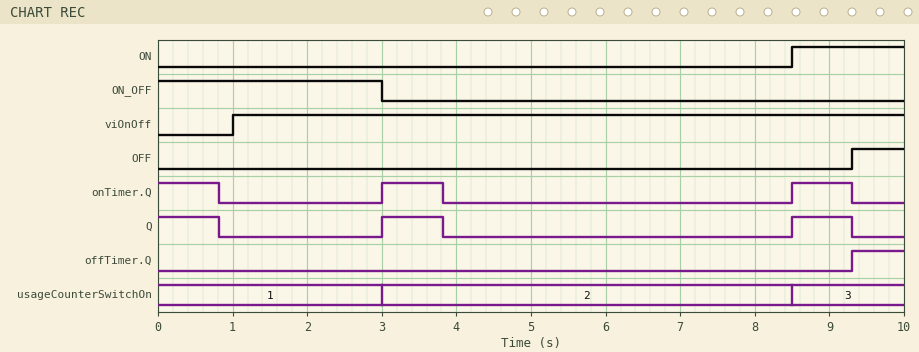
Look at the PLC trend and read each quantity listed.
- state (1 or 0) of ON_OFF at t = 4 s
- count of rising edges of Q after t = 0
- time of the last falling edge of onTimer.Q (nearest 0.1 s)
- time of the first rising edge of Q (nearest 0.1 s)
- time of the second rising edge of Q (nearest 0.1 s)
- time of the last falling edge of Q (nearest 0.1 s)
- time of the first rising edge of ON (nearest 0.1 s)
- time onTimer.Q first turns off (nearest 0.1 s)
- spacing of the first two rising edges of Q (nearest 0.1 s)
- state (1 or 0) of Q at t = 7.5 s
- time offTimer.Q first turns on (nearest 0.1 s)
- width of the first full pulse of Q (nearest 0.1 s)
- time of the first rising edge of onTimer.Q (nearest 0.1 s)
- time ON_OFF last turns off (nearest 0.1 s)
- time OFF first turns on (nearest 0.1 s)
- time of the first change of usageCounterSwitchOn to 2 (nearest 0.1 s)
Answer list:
0
2
9.3 s
3.0 s
8.5 s
9.3 s
8.5 s
0.8 s
5.5 s
0
9.3 s
0.8 s
3.0 s
3.0 s
9.3 s
3.0 s
